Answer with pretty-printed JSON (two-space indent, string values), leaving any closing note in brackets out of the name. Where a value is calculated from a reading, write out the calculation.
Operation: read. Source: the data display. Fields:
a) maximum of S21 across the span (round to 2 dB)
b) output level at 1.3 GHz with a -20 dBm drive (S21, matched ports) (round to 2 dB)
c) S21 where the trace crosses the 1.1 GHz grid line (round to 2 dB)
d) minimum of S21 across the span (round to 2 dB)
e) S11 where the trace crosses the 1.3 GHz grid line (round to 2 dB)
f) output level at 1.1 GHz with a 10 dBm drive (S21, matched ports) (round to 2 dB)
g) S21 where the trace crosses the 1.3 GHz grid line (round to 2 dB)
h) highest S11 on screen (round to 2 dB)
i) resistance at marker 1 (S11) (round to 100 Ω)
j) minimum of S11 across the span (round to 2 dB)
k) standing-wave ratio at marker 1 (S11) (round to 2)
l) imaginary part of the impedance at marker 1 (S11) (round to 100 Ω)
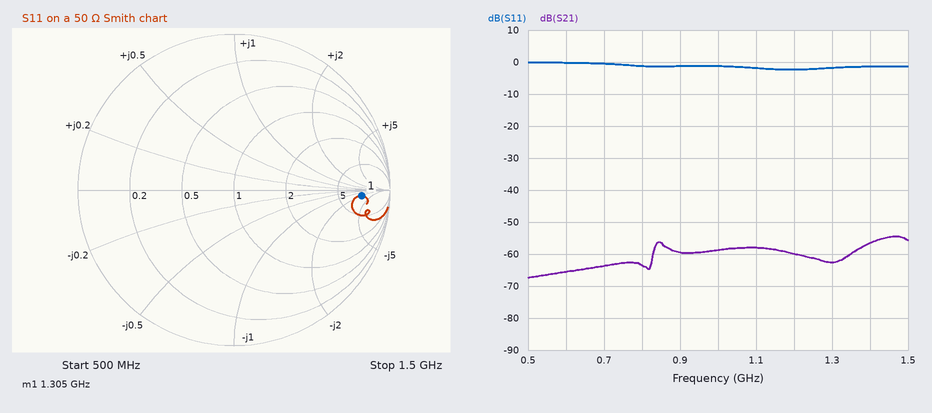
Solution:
{
  "maximum of S21 across the span": "-54 dB",
  "output level at 1.3 GHz with a -20 dBm drive (S21, matched ports)": "-20 dBm + (-62 dB) = -82 dBm",
  "S21 where the trace crosses the 1.1 GHz grid line": "-58 dB",
  "minimum of S21 across the span": "-68 dB",
  "S11 where the trace crosses the 1.3 GHz grid line": "-2 dB",
  "output level at 1.1 GHz with a 10 dBm drive (S21, matched ports)": "10 dBm + (-58 dB) = -48 dBm",
  "S21 where the trace crosses the 1.3 GHz grid line": "-62 dB",
  "highest S11 on screen": "0 dB",
  "resistance at marker 1 (S11)": "500 Ω",
  "minimum of S11 across the span": "-2 dB",
  "standing-wave ratio at marker 1 (S11)": "10",
  "imaginary part of the impedance at marker 1 (S11)": "-100 Ω"
}
